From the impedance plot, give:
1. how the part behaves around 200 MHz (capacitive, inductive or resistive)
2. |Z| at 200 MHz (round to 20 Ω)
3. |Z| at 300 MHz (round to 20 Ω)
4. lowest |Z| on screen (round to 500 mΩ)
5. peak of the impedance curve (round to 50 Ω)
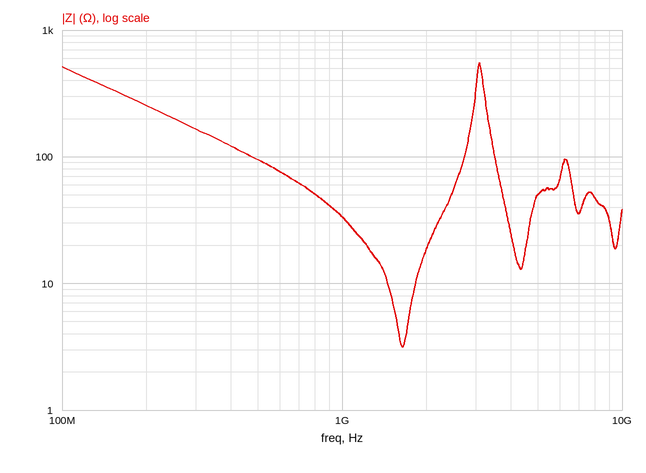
capacitive
260 Ω
160 Ω
3.0 Ω
550 Ω
